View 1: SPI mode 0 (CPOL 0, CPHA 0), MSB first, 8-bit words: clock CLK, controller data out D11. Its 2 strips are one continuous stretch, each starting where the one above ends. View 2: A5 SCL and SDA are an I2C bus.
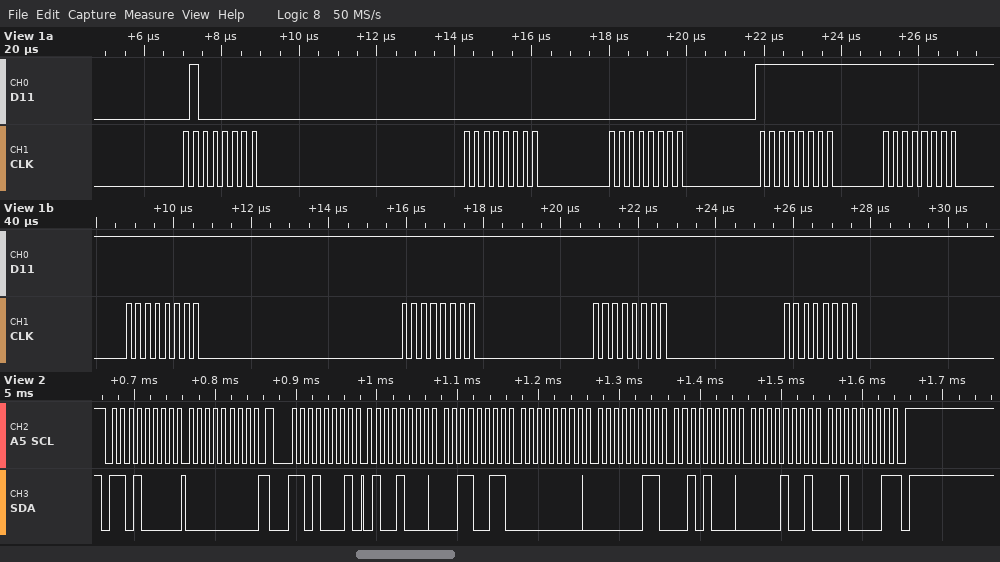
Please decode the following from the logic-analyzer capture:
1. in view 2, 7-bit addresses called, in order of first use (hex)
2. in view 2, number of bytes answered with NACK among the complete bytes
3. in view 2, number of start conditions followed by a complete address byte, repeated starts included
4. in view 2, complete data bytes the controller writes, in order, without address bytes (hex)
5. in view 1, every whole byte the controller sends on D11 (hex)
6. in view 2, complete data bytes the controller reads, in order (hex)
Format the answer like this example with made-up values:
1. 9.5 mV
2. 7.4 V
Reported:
1. 0x68
2. 1
3. 2
4. 00
5. 0x40 0x00 0x00 0xFF 0xFF 0xFF 0xFF 0xFF 0xFF
6. 48 33 00 03 28 09 21
